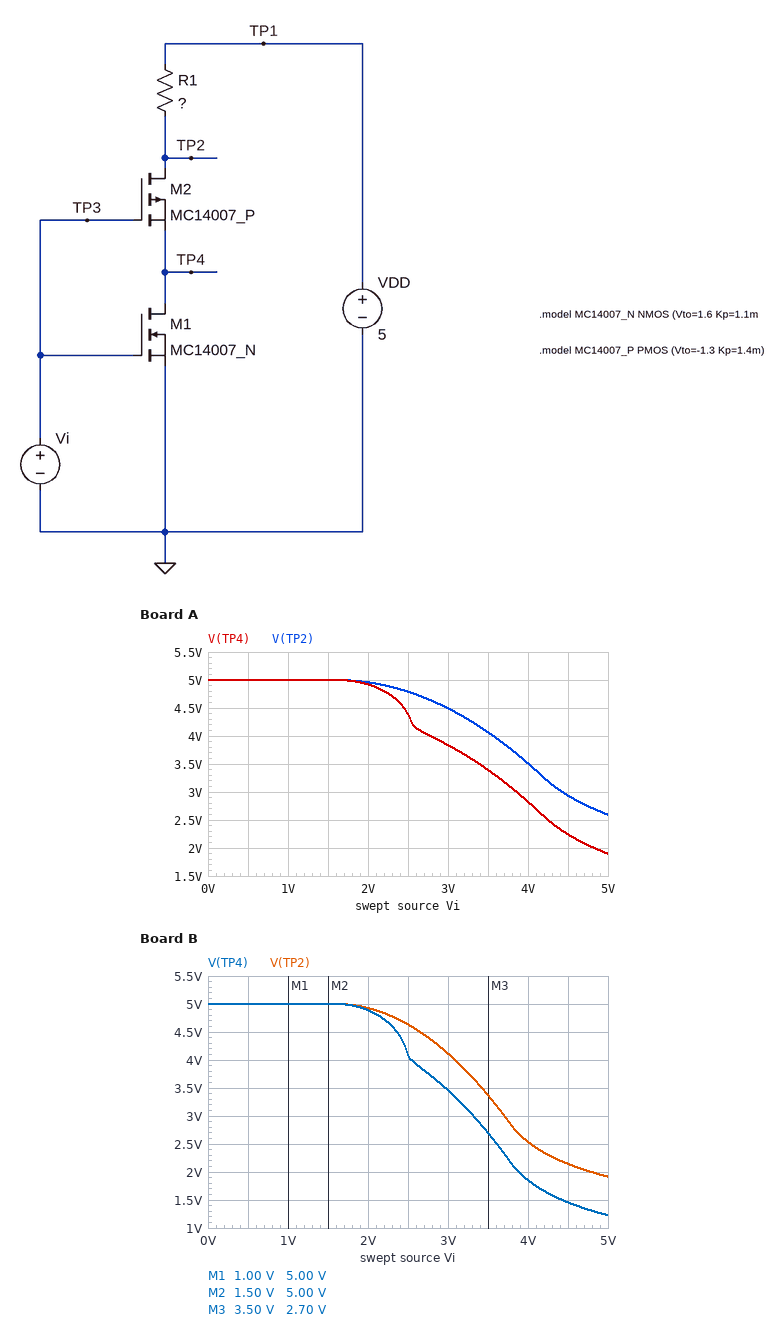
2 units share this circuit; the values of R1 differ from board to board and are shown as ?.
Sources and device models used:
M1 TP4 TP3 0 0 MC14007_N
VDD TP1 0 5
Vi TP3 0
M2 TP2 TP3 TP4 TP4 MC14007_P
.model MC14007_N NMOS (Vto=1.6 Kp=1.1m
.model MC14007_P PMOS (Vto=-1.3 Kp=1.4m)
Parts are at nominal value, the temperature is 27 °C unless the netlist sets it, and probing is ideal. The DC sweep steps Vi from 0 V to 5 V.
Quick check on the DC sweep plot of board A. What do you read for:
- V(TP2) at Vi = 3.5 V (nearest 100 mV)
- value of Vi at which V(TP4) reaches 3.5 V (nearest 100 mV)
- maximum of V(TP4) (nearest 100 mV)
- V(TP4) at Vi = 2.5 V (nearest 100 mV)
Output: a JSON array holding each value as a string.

["4.1 V", "3.4 V", "5.0 V", "4.4 V"]
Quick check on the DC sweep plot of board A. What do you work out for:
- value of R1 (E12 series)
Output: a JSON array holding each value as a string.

["470 Ω"]
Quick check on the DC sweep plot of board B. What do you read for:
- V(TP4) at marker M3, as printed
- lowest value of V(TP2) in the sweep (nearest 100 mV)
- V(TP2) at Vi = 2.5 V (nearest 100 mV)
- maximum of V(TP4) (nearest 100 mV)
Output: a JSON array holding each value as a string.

["2.70 V", "1.9 V", "4.6 V", "5.0 V"]
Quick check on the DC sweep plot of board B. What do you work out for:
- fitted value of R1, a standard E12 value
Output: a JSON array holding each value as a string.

["820 Ω"]
